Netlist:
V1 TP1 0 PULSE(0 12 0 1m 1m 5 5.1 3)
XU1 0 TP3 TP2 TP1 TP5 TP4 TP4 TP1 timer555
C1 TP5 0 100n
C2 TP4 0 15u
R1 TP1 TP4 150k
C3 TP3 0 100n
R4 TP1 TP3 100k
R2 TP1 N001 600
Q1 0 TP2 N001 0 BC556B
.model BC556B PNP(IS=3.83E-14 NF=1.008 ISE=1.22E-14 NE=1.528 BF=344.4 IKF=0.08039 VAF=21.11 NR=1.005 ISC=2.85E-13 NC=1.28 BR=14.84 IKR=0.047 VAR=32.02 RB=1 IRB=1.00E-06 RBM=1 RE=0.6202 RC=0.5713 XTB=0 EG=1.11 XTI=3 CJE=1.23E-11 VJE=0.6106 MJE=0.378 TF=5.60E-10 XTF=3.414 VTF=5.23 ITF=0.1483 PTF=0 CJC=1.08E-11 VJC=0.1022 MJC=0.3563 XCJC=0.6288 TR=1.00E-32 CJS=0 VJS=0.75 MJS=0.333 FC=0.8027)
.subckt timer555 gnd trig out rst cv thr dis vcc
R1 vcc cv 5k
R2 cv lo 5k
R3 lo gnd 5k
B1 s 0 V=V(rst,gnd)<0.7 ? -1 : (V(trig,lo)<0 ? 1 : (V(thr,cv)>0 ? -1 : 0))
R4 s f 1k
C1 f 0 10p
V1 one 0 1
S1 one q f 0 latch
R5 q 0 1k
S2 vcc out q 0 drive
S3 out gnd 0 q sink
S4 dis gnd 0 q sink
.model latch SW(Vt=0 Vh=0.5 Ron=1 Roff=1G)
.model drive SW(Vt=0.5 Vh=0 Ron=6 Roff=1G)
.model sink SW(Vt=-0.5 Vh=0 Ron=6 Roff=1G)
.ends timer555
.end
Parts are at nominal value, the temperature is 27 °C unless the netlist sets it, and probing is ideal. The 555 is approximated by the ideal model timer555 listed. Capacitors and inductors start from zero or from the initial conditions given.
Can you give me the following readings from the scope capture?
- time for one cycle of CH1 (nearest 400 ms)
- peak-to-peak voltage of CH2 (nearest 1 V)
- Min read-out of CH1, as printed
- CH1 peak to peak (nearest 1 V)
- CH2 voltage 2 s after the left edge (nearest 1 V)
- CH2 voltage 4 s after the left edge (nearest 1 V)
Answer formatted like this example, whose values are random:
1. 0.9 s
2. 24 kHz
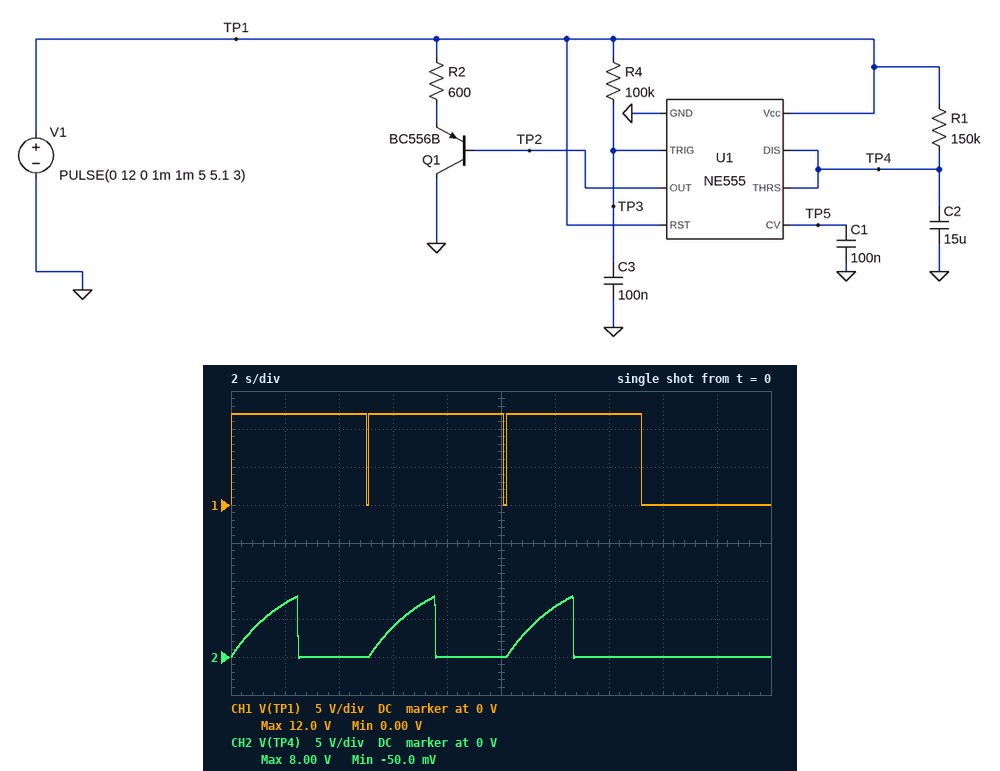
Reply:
1. 5.2 s
2. 8 V
3. 0.00 V
4. 12 V
5. 7 V
6. 0 V
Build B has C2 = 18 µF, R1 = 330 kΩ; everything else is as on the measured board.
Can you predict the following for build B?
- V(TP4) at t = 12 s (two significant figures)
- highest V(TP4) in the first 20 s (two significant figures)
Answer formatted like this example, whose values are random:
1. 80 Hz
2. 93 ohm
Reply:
1. 3.1 V
2. 6.8 V
